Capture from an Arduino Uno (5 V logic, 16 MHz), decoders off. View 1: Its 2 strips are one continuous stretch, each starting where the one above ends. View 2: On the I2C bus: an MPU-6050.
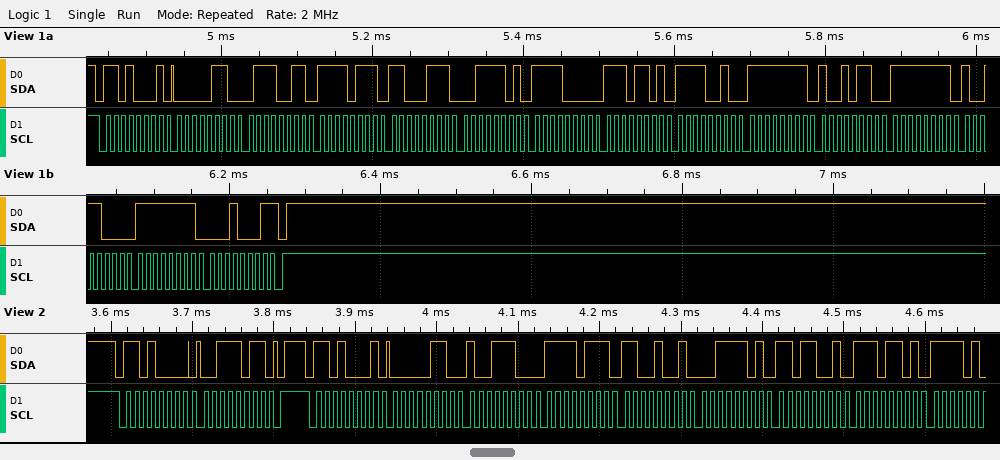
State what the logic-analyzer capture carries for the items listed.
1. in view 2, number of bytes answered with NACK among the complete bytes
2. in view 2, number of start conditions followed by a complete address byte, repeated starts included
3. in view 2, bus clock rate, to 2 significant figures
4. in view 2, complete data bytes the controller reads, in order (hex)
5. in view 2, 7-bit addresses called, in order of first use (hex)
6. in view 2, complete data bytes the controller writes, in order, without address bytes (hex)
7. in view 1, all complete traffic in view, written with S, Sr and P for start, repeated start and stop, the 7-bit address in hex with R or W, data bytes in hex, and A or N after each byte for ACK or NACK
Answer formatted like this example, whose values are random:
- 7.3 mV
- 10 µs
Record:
- 0
- 2
- 100 kHz
- 06 9C F7 C9 3D D9 ED
- 0x68
- 3B
- S 68R A 06 A 73 A F7 A C7 A 3D A F0 A ED A F2 A FF A 96 A FF A 98 A FF A 11 N P
